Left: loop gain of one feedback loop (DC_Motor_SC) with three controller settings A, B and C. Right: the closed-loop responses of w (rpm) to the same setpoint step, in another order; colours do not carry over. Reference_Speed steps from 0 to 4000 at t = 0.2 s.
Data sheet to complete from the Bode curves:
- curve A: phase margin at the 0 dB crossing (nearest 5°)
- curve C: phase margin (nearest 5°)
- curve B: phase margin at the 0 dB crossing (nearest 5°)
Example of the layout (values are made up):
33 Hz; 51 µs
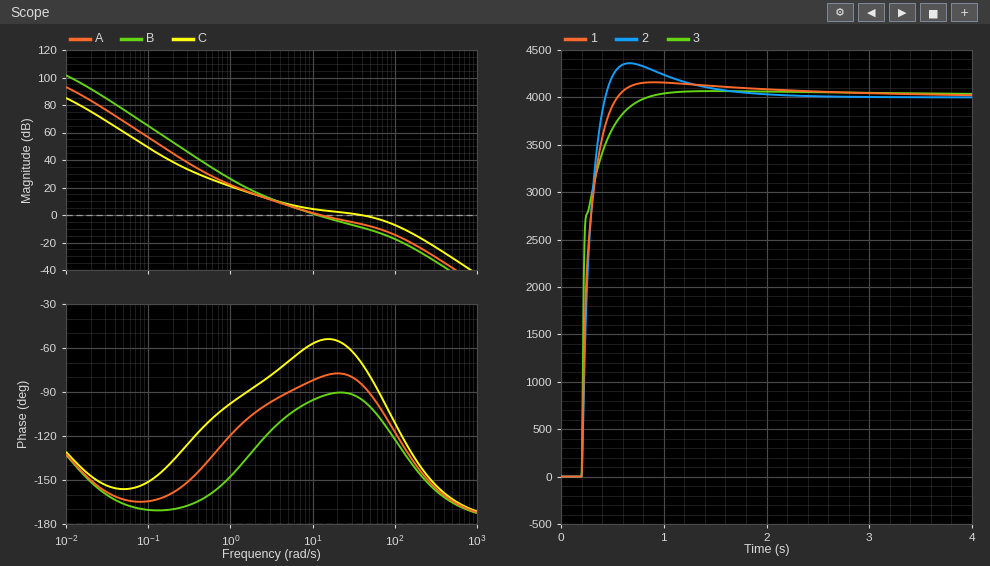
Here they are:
100°; 110°; 85°
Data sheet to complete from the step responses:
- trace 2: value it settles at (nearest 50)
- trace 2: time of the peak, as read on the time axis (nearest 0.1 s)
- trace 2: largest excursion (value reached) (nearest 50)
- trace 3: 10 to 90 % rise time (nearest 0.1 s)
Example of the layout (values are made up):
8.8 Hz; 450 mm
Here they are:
4000; 0.7 s; 4350; 0.3 s
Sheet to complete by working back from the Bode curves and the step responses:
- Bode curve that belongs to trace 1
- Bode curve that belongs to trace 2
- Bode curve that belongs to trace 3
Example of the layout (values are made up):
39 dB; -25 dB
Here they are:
A; B; C
